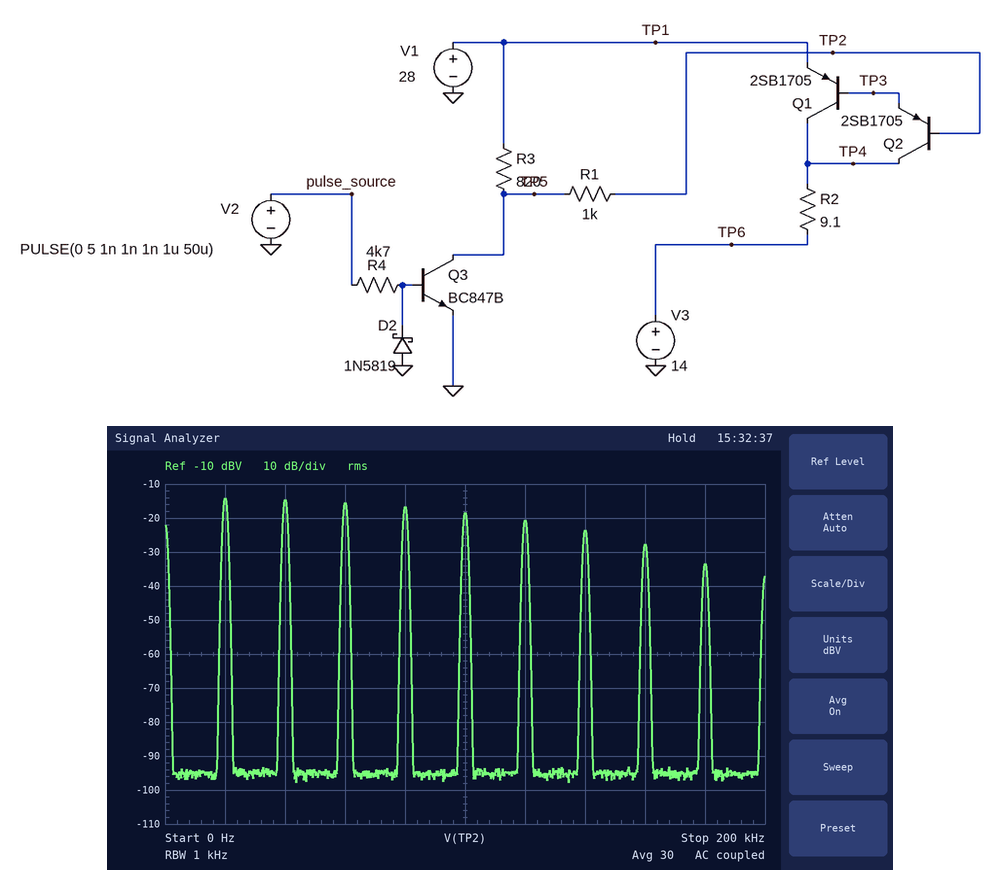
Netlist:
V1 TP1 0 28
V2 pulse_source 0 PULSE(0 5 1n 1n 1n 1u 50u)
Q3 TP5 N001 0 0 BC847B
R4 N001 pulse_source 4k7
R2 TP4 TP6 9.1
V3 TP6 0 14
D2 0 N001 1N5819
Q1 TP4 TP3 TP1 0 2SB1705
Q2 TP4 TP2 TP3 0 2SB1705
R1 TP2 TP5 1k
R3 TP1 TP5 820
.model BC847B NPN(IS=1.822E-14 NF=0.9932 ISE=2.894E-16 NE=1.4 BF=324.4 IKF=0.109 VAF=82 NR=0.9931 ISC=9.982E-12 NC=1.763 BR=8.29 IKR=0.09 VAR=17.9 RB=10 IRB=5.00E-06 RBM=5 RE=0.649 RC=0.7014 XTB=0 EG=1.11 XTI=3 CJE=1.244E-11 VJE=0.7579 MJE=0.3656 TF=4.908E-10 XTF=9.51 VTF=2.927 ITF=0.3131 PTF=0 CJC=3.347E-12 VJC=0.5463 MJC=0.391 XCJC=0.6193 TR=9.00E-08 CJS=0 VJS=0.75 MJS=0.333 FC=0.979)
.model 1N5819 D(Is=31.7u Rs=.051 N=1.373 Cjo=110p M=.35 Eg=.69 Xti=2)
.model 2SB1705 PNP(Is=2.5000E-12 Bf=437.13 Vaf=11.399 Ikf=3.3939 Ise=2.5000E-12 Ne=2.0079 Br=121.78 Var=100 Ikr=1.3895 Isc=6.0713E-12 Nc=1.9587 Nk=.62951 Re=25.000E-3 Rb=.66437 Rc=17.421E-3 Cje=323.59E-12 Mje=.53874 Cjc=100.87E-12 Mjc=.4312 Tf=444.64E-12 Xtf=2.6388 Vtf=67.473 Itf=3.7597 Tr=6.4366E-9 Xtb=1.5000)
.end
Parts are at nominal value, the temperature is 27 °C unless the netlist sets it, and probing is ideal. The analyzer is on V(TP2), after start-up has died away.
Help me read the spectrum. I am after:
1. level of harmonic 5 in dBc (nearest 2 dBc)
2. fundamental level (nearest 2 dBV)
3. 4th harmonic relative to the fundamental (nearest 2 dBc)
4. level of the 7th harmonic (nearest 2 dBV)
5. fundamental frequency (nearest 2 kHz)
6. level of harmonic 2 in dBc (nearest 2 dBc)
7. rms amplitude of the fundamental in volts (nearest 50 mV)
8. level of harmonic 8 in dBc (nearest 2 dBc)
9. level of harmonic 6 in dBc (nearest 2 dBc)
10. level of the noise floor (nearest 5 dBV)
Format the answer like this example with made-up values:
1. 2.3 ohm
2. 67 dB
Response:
1. -4 dBc
2. -14 dBV
3. -2 dBc
4. -24 dBV
5. 20 kHz
6. 0 dBc
7. 200 mV
8. -14 dBc
9. -6 dBc
10. -95 dBV
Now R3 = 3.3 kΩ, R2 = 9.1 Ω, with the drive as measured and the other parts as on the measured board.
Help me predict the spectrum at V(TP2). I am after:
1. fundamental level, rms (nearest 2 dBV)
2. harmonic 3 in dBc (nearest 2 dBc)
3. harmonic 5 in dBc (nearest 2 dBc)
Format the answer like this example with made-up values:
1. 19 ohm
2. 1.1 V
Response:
1. -10 dBV
2. -4 dBc
3. -12 dBc
